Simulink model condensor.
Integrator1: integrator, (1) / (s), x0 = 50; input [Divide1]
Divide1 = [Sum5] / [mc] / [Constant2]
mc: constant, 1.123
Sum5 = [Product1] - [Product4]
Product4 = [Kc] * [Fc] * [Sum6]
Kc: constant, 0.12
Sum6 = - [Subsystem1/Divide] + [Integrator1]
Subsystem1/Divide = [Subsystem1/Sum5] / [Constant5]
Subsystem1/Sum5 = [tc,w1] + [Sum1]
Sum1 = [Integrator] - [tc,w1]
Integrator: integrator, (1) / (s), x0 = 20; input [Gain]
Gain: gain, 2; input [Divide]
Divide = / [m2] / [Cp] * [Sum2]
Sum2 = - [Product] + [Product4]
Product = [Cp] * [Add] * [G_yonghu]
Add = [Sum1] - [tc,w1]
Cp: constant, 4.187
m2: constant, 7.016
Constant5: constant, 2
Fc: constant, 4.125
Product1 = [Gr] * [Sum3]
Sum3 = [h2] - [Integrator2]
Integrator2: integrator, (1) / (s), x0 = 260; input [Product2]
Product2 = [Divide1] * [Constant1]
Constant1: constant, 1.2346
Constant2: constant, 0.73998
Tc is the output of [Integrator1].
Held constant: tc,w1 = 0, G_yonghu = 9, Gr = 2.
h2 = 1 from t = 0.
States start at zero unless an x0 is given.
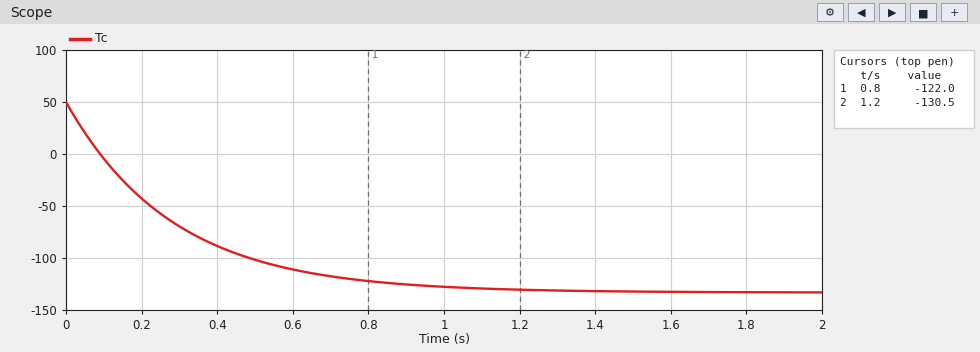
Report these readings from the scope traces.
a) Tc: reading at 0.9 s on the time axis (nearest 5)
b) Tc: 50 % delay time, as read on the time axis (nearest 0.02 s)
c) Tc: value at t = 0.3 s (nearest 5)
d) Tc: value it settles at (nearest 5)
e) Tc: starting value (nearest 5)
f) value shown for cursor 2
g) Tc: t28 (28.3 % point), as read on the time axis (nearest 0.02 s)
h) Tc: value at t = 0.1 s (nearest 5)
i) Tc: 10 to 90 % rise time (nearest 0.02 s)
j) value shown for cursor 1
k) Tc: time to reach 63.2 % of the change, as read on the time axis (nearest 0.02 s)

-125
0.20 s
-70
-135
50
-130.5
0.10 s
-5
0.62 s
-122.0
0.28 s
